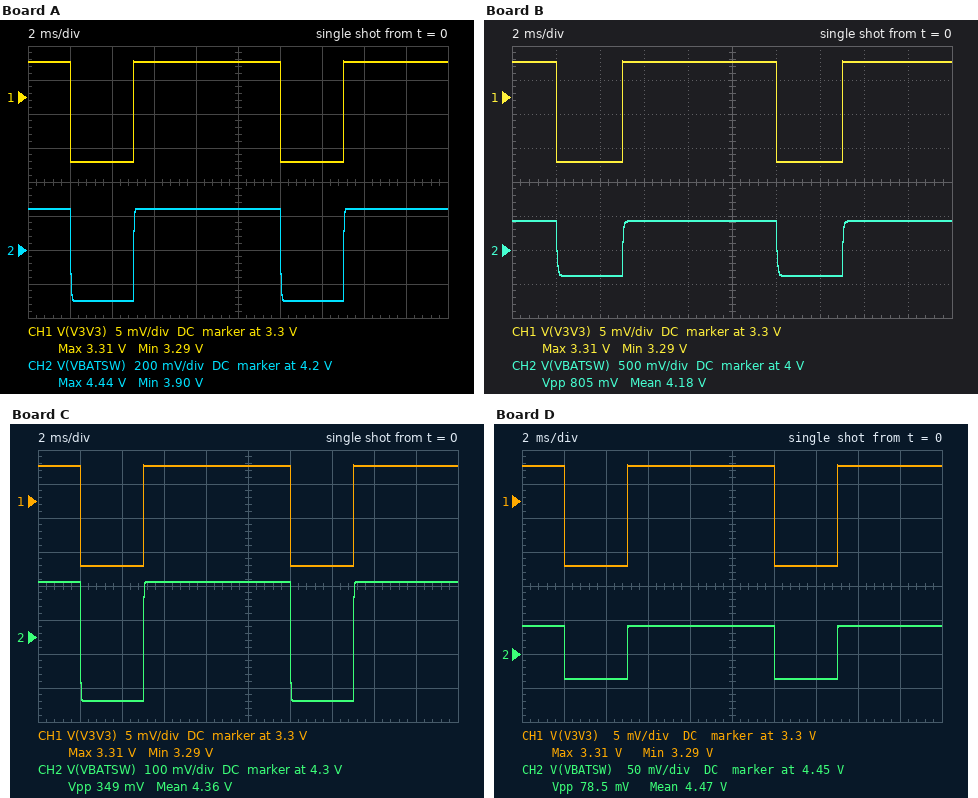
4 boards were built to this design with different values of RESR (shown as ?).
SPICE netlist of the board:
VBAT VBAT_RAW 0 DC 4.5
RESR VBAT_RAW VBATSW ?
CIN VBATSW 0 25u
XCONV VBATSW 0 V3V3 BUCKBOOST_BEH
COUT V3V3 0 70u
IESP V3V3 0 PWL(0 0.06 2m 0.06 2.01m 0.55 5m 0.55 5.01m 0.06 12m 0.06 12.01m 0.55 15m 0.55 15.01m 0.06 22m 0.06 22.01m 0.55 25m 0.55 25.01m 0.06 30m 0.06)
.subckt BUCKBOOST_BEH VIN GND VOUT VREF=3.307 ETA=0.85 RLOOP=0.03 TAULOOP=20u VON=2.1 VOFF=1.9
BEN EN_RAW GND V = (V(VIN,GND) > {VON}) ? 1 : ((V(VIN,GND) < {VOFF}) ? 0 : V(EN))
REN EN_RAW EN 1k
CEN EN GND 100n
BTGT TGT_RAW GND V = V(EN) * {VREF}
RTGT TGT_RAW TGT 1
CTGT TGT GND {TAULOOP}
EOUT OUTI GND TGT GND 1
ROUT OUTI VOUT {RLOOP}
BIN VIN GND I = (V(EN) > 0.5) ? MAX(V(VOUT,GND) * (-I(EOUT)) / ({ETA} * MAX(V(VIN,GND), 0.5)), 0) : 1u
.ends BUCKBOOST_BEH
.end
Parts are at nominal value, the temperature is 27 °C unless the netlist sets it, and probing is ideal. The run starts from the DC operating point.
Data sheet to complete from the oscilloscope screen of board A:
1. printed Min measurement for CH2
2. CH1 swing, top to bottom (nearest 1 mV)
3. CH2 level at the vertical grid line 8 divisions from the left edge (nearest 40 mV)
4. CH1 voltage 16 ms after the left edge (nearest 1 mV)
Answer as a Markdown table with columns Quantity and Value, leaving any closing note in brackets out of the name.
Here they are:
| Quantity | Value |
|---|---|
| printed Min measurement for CH2 | 3.90 V |
| CH1 swing, top to bottom | 15 mV |
| CH2 level at the vertical grid line 8 divisions from the left edge | 4.44 V |
| CH1 voltage 16 ms after the left edge | 3.305 V |
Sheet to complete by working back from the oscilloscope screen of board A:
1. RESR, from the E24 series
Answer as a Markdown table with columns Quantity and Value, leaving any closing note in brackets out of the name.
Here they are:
| Quantity | Value |
|---|---|
| RESR, from the E24 series | 1.1 Ω |
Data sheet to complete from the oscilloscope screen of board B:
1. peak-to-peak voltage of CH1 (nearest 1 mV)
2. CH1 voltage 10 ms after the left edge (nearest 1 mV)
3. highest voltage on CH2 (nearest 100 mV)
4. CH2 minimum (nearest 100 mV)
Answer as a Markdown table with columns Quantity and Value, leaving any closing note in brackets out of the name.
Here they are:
| Quantity | Value |
|---|---|
| peak-to-peak voltage of CH1 | 15 mV |
| CH1 voltage 10 ms after the left edge | 3.305 V |
| highest voltage on CH2 | 4.4 V |
| CH2 minimum | 3.6 V |
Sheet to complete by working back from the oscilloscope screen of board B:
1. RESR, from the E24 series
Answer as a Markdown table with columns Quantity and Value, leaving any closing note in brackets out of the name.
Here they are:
| Quantity | Value |
|---|---|
| RESR, from the E24 series | 1.5 Ω |
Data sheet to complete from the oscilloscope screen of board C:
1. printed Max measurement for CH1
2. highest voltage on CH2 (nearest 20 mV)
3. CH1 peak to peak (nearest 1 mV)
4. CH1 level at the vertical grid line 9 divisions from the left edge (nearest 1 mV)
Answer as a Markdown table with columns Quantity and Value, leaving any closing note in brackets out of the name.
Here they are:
| Quantity | Value |
|---|---|
| printed Max measurement for CH1 | 3.31 V |
| highest voltage on CH2 | 4.46 V |
| CH1 peak to peak | 15 mV |
| CH1 level at the vertical grid line 9 divisions from the left edge | 3.305 V |
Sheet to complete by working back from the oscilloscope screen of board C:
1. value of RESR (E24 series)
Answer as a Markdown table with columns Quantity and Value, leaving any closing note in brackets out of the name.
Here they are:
| Quantity | Value |
|---|---|
| value of RESR | 0.75 Ω |
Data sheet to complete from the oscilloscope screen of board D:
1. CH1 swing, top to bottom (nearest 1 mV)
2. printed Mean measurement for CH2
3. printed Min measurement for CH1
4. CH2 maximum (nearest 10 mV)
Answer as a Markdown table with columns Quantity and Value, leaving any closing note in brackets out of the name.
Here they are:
| Quantity | Value |
|---|---|
| CH1 swing, top to bottom | 15 mV |
| printed Mean measurement for CH2 | 4.47 V |
| printed Min measurement for CH1 | 3.29 V |
| CH2 maximum | 4.49 V |
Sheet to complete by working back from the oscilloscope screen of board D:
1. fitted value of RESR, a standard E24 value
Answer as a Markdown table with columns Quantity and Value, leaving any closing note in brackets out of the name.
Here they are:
| Quantity | Value |
|---|---|
| fitted value of RESR, a standard E24 value | 0.18 Ω |
